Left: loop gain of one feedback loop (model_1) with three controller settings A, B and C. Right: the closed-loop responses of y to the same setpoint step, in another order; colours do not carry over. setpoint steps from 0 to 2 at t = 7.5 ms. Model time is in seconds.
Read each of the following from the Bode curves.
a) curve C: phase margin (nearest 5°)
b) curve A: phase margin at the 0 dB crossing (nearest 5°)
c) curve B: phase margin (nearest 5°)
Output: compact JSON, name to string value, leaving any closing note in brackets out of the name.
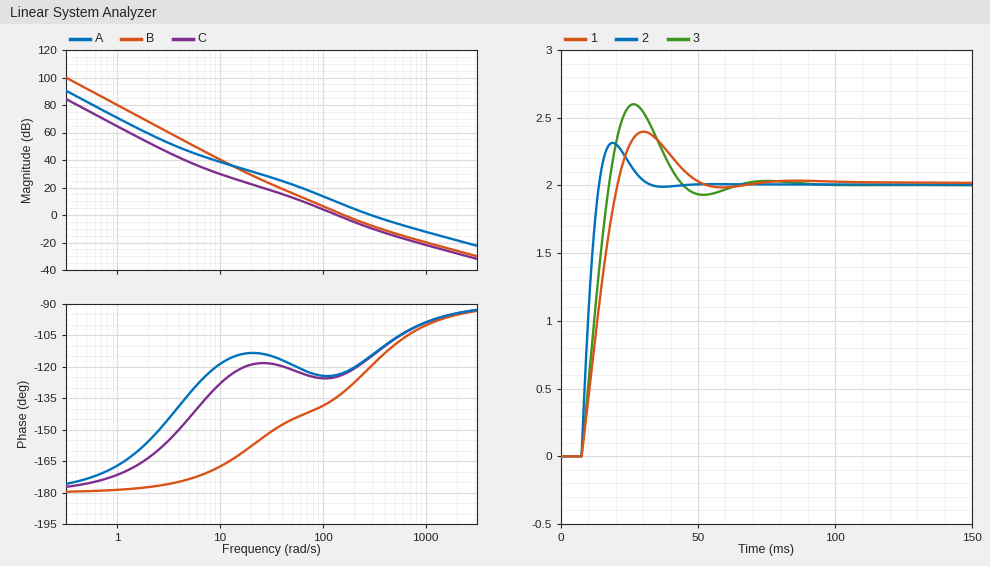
{"curve C: phase margin": "55°", "curve A: phase margin at the 0 dB crossing": "65°", "curve B: phase margin": "50°"}
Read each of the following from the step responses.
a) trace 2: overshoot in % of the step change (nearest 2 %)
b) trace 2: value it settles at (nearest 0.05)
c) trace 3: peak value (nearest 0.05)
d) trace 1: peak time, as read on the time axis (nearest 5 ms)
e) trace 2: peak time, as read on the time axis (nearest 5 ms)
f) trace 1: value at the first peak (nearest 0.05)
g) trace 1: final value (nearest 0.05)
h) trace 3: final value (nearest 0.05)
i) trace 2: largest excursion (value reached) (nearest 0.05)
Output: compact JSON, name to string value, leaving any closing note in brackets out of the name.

{"trace 2: overshoot in % of the step change": "16 %", "trace 2: value it settles at": "2.00", "trace 3: peak value": "2.60", "trace 1: peak time, as read on the time axis": "30 ms", "trace 2: peak time, as read on the time axis": "20 ms", "trace 1: value at the first peak": "2.40", "trace 1: final value": "2.00", "trace 3: final value": "2.00", "trace 2: largest excursion (value reached)": "2.30"}
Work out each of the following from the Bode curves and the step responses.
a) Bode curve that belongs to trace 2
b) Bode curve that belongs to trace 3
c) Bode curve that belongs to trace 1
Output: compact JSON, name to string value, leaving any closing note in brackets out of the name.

{"Bode curve that belongs to trace 2": "A", "Bode curve that belongs to trace 3": "B", "Bode curve that belongs to trace 1": "C"}
